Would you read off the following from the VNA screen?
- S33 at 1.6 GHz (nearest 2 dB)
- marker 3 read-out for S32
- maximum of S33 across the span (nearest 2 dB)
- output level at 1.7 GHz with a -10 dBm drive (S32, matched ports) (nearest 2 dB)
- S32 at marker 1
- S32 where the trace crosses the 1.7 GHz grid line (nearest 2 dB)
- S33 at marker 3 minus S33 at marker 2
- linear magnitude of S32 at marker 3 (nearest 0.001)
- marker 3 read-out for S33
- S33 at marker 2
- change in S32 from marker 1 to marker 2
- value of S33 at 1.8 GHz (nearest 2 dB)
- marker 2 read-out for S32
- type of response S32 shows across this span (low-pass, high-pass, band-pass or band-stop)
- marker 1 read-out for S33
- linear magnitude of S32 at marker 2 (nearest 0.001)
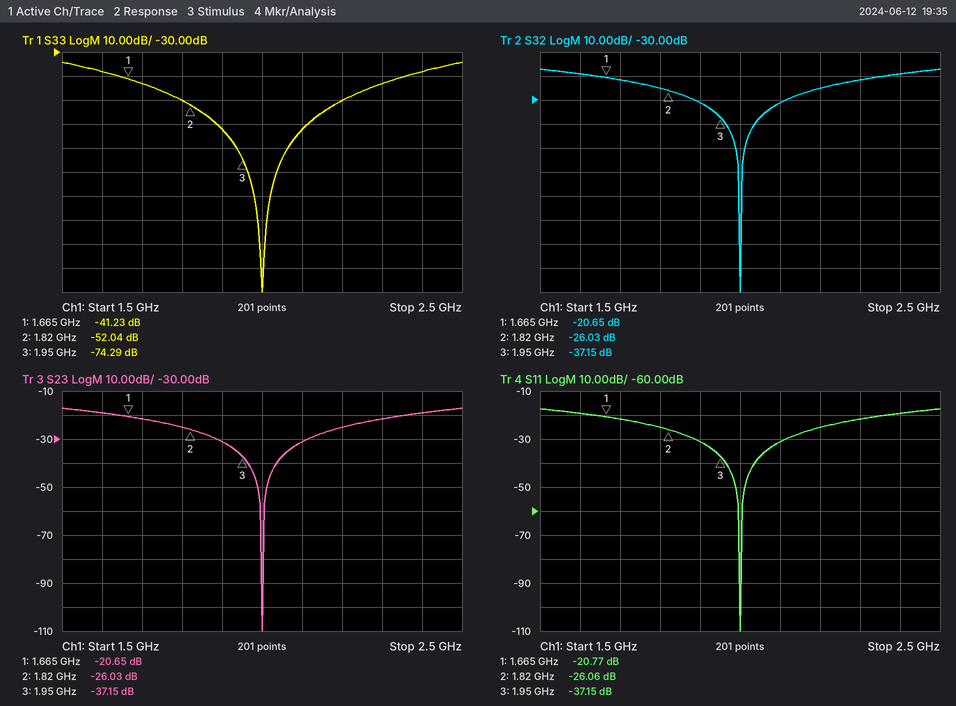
-38 dB
-37.15 dB
-34 dB
-32 dBm
-20.65 dB
-22 dB
-22.25 dB
0.014
-74.29 dB
-52.04 dB
-5.38 dB
-50 dB
-26.03 dB
band-stop
-41.23 dB
0.050
